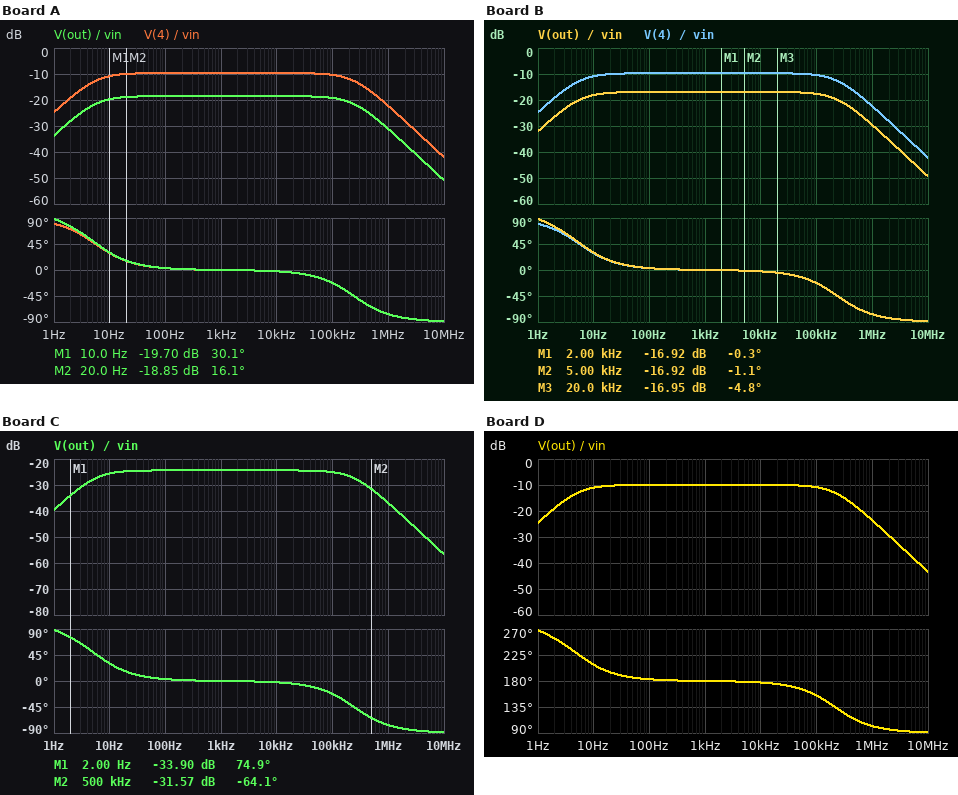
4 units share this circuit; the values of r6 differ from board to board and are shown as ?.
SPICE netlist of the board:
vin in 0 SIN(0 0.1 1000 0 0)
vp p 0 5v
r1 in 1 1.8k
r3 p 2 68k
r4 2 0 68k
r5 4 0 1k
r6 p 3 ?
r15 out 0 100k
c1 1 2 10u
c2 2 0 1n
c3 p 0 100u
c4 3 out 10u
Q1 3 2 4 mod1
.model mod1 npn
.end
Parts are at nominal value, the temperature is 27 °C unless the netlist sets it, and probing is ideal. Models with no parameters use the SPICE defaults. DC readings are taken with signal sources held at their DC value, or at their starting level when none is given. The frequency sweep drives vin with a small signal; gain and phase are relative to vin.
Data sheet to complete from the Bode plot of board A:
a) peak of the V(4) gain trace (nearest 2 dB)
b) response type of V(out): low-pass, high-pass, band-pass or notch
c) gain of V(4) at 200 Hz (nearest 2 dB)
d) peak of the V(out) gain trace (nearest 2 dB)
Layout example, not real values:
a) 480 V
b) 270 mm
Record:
a) -10 dB
b) band-pass
c) -10 dB
d) -18 dB
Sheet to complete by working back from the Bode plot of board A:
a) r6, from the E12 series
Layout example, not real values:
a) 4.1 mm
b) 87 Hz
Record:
a) 12 kΩ
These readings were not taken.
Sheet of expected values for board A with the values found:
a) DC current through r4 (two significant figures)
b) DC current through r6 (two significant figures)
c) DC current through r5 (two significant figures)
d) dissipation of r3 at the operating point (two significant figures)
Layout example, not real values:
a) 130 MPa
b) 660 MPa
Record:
a) 17 µA
b) 380 µA
c) 420 µA
d) 220 µW
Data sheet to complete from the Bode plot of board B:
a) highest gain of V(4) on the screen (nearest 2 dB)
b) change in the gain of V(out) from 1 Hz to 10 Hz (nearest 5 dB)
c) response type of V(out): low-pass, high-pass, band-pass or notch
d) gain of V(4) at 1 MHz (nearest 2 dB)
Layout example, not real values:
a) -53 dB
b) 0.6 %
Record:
a) -10 dB
b) 15 dB
c) band-pass
d) -22 dB
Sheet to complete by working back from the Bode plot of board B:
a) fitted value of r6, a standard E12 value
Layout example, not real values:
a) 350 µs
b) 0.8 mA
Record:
a) 15 kΩ
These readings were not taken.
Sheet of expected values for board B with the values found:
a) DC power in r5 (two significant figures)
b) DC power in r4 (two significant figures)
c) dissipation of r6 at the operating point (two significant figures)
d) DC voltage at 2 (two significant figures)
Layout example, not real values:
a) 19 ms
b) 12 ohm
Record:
a) 120 µW
b) 18 µW
c) 1.4 mW
d) 1.1 V
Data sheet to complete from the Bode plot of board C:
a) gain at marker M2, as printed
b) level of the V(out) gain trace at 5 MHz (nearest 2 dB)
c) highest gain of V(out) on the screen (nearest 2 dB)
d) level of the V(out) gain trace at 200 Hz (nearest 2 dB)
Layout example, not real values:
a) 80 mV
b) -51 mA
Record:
a) -31.57 dB
b) -50 dB
c) -24 dB
d) -24 dB
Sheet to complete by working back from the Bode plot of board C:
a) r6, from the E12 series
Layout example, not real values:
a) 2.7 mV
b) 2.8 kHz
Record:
a) 8.2 kΩ
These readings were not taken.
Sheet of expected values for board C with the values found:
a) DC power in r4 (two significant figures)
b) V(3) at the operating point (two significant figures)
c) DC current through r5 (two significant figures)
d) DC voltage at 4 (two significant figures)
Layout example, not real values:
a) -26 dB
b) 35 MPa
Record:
a) 26 µW
b) 640 mV
c) 570 µA
d) 570 mV
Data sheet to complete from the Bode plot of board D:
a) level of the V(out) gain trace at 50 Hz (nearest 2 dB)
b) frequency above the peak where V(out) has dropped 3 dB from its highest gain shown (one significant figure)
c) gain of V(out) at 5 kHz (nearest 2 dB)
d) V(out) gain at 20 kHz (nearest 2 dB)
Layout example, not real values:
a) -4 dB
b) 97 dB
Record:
a) -10 dB
b) 200 kHz
c) -10 dB
d) -10 dB
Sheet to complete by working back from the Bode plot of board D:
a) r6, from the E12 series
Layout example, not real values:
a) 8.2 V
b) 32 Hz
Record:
a) 3.9 kΩ
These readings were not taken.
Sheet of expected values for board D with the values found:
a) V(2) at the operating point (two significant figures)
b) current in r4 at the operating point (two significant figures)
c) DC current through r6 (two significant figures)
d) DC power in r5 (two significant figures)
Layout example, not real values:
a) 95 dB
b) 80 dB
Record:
a) 1.8 V
b) 26 µA
c) 990 µA
d) 1.0 mW
